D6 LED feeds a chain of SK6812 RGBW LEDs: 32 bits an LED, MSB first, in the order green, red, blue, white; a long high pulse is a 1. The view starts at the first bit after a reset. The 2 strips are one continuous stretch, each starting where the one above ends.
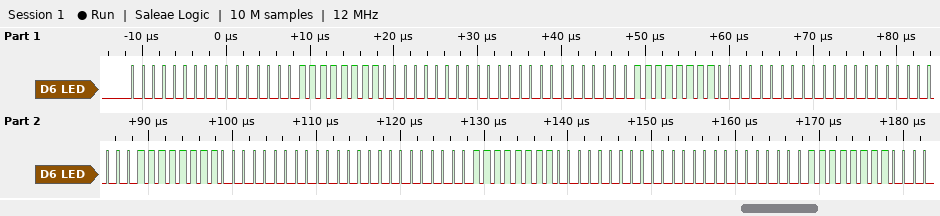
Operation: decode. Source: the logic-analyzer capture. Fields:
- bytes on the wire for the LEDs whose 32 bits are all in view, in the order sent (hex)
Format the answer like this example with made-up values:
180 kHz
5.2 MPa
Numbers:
00 00 FF 00 00 00 FF 00 00 00 FF 00 00 00 FF 00
